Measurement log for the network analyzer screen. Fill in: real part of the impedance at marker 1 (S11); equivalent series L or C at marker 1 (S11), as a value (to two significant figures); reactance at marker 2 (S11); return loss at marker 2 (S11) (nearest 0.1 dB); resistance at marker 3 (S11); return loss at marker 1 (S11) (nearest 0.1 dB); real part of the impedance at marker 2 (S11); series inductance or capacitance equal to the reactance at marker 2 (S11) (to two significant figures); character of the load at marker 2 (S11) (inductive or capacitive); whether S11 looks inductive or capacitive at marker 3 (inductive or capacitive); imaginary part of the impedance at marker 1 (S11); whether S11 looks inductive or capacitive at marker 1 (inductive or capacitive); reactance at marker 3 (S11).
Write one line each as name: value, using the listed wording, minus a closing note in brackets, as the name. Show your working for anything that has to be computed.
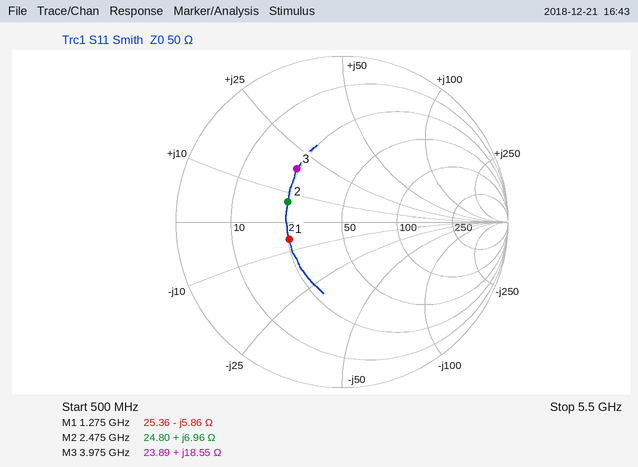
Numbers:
real part of the impedance at marker 1: 25.36 Ω
equivalent series L or C at marker 1 (S11), as a value: C = 1/(2π × 1.275 GHz × 5.86 Ω) ≈ 21 pF
reactance at marker 2: +6.96 Ω
return loss at marker 2 (S11): 9.2 dB
resistance at marker 3: 23.89 Ω
return loss at marker 1 (S11): 9.5 dB
real part of the impedance at marker 2: 24.80 Ω
series inductance or capacitance equal to the reactance at marker 2 (S11): L = 6.96 Ω/(2π × 2.475 GHz) ≈ 448 pH, so 450 pH to two significant figures
character of the load at marker 2 (S11): inductive
whether S11 looks inductive or capacitive at marker 3: inductive
imaginary part of the impedance at marker 1: -5.86 Ω
whether S11 looks inductive or capacitive at marker 1: capacitive
reactance at marker 3: +18.55 Ω
